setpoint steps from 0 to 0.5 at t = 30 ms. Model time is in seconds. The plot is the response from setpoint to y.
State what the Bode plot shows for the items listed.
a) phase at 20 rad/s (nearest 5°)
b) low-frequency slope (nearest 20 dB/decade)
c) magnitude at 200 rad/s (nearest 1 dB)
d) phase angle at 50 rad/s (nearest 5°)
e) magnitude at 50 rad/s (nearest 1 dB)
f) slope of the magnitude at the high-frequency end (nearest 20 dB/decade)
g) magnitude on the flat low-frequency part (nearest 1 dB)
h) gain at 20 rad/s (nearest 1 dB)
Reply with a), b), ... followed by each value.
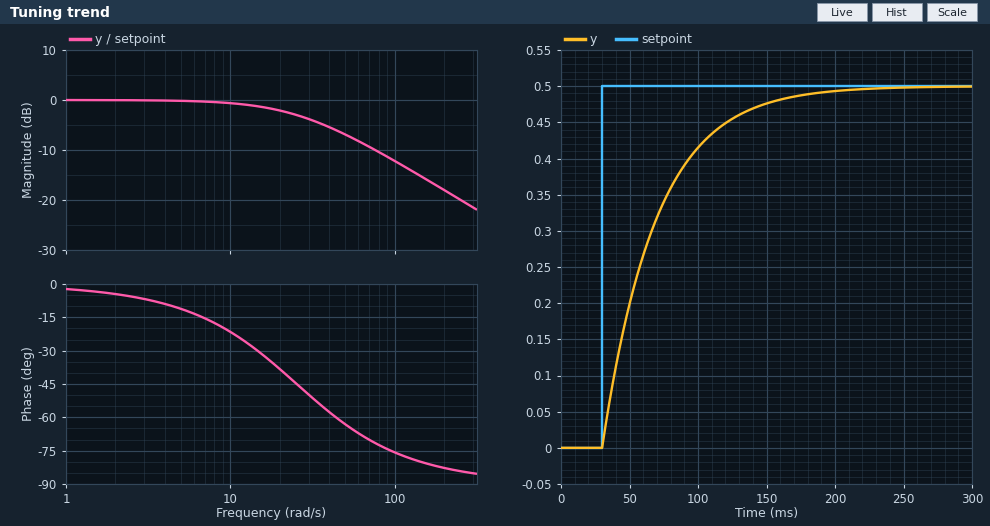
a) -40°
b) 0 dB/decade
c) -18 dB
d) -65°
e) -7 dB
f) -20 dB/decade
g) 0 dB
h) -2 dB
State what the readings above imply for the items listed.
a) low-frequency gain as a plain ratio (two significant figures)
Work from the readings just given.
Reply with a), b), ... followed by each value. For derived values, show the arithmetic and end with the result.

a) 10^(0 / 20) = 1.0
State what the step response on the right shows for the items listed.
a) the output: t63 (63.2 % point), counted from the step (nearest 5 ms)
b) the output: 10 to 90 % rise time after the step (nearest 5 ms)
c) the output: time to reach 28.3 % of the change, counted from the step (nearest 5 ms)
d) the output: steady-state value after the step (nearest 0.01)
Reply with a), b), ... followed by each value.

a) 40 ms
b) 85 ms
c) 15 ms
d) 0.50
